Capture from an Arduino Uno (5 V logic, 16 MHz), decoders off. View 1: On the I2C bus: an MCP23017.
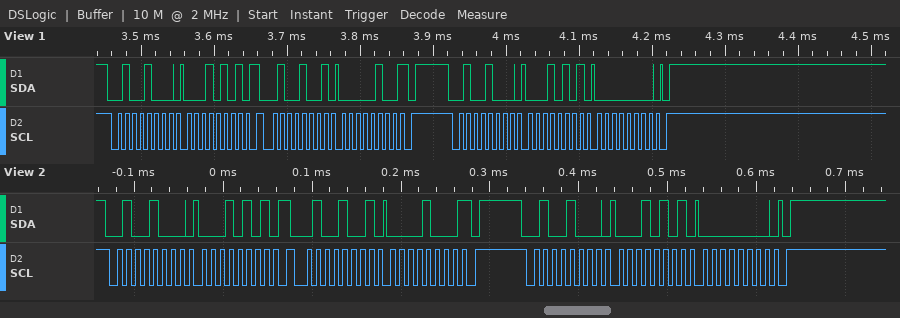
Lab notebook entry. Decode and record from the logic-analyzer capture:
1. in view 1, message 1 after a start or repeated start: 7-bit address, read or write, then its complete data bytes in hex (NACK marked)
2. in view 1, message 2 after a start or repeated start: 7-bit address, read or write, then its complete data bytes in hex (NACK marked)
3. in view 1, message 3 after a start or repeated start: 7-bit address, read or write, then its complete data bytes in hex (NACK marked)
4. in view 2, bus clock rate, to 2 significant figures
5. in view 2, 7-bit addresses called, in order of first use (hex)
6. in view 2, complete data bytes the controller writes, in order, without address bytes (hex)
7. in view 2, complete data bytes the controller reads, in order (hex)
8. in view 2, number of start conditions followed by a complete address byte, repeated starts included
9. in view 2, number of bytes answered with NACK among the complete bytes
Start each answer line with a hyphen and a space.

- 0x24 write: 15
- 0x24 read: 04 NACK
- 0x24 write: 15 00
- 100 kHz
- 0x24
- 15 15 00
- 08
- 3
- 1
